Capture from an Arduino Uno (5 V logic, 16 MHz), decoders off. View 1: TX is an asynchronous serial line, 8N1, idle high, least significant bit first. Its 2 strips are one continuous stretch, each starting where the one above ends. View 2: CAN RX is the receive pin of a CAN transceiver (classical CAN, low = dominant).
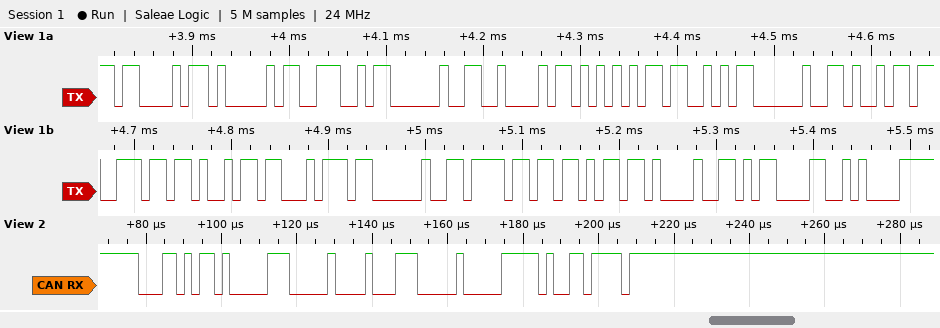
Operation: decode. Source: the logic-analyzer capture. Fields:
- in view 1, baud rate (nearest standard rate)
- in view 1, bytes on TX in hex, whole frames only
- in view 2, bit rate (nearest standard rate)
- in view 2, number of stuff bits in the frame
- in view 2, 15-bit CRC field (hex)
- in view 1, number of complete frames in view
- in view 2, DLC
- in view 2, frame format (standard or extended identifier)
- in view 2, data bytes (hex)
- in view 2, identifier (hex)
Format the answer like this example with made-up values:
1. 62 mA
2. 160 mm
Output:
1. 115200 baud
2. 43 41 4E 20 42 55 53 20 69 6E 69 74 20 6F 6B 21 0D 0A
3. 500 kbit/s
4. 5
5. 0x1F37
6. 18
7. 3
8. standard
9. 00 47 00
10. 0x1AD
